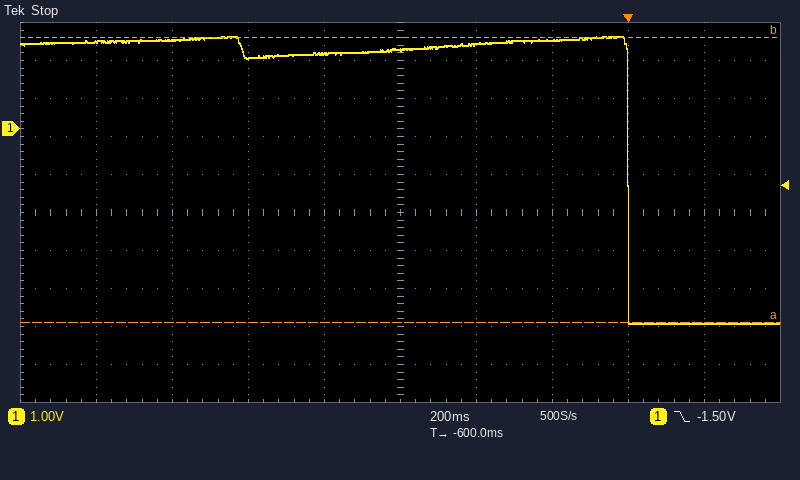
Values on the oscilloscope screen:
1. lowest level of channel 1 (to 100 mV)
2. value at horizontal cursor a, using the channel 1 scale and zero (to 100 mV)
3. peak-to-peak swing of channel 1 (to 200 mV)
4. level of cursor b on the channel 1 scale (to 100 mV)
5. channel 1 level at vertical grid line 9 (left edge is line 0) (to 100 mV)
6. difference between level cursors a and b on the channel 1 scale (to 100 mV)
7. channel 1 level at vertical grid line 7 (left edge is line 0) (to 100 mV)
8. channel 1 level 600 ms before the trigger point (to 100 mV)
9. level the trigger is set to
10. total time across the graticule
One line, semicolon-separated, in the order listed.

-5.1 V; -5.1 V; 7.6 V; 2.4 V; -5.1 V; 7.5 V; 2.3 V; 2.1 V; -1.50 V; 2 s
